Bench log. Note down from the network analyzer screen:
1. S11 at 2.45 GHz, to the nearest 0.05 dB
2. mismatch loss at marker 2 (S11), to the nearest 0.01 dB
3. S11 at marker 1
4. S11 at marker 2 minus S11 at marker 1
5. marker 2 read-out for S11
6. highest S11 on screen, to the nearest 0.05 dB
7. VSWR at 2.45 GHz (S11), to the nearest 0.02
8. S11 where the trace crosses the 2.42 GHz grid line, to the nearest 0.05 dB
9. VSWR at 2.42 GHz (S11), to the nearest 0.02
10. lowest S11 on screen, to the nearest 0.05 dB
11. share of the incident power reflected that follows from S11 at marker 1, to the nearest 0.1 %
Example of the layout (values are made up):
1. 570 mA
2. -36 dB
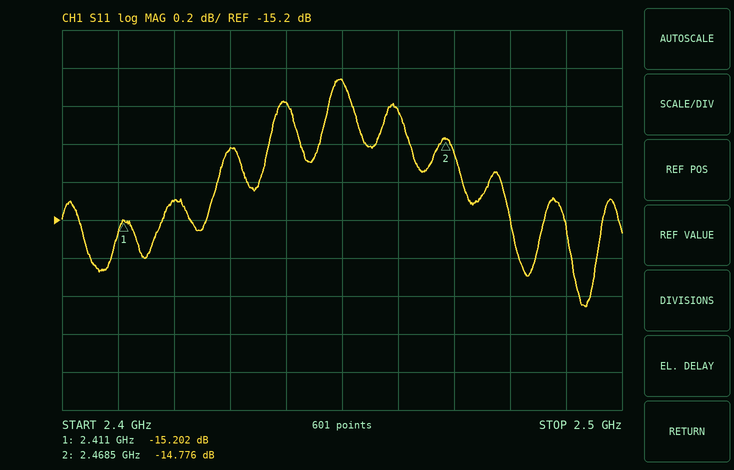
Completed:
1. -14.45 dB
2. 0.15 dB
3. -15.202 dB
4. 0.426 dB
5. -14.776 dB
6. -14.45 dB
7. 1.46
8. -15.10 dB
9. 1.42
10. -15.65 dB
11. 3.0 %
